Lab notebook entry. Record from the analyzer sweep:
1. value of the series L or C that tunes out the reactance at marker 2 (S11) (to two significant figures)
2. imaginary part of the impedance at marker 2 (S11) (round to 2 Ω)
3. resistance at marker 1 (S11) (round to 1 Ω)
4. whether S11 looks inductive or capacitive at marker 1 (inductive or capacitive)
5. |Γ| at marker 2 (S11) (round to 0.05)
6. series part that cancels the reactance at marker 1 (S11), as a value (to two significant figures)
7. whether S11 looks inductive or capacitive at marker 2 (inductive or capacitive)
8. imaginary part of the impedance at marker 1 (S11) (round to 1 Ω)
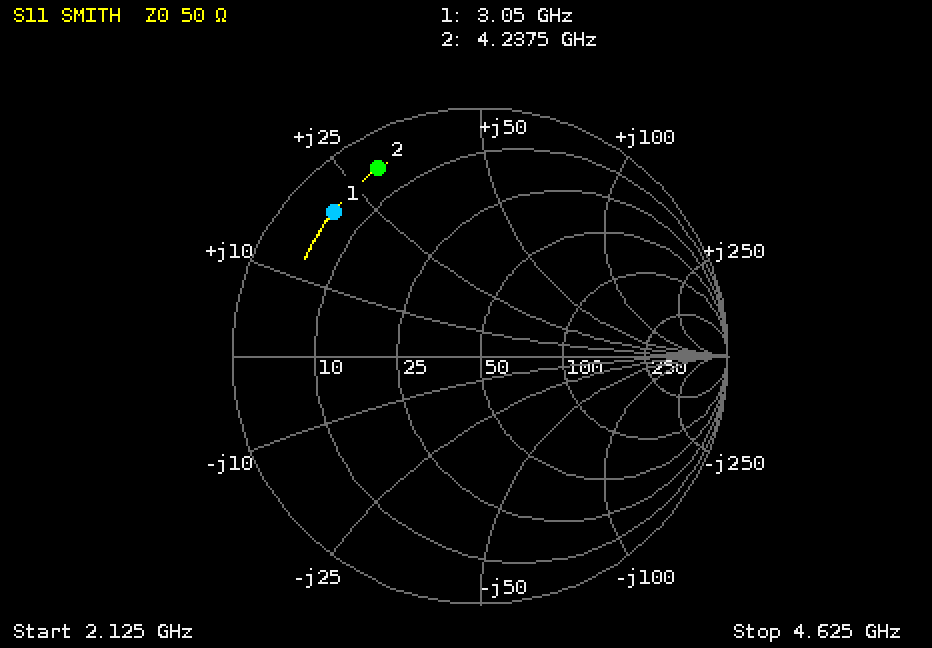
1.3 pF
+30 Ω
5 Ω
inductive
0.85
2.6 pF
inductive
+20 Ω
